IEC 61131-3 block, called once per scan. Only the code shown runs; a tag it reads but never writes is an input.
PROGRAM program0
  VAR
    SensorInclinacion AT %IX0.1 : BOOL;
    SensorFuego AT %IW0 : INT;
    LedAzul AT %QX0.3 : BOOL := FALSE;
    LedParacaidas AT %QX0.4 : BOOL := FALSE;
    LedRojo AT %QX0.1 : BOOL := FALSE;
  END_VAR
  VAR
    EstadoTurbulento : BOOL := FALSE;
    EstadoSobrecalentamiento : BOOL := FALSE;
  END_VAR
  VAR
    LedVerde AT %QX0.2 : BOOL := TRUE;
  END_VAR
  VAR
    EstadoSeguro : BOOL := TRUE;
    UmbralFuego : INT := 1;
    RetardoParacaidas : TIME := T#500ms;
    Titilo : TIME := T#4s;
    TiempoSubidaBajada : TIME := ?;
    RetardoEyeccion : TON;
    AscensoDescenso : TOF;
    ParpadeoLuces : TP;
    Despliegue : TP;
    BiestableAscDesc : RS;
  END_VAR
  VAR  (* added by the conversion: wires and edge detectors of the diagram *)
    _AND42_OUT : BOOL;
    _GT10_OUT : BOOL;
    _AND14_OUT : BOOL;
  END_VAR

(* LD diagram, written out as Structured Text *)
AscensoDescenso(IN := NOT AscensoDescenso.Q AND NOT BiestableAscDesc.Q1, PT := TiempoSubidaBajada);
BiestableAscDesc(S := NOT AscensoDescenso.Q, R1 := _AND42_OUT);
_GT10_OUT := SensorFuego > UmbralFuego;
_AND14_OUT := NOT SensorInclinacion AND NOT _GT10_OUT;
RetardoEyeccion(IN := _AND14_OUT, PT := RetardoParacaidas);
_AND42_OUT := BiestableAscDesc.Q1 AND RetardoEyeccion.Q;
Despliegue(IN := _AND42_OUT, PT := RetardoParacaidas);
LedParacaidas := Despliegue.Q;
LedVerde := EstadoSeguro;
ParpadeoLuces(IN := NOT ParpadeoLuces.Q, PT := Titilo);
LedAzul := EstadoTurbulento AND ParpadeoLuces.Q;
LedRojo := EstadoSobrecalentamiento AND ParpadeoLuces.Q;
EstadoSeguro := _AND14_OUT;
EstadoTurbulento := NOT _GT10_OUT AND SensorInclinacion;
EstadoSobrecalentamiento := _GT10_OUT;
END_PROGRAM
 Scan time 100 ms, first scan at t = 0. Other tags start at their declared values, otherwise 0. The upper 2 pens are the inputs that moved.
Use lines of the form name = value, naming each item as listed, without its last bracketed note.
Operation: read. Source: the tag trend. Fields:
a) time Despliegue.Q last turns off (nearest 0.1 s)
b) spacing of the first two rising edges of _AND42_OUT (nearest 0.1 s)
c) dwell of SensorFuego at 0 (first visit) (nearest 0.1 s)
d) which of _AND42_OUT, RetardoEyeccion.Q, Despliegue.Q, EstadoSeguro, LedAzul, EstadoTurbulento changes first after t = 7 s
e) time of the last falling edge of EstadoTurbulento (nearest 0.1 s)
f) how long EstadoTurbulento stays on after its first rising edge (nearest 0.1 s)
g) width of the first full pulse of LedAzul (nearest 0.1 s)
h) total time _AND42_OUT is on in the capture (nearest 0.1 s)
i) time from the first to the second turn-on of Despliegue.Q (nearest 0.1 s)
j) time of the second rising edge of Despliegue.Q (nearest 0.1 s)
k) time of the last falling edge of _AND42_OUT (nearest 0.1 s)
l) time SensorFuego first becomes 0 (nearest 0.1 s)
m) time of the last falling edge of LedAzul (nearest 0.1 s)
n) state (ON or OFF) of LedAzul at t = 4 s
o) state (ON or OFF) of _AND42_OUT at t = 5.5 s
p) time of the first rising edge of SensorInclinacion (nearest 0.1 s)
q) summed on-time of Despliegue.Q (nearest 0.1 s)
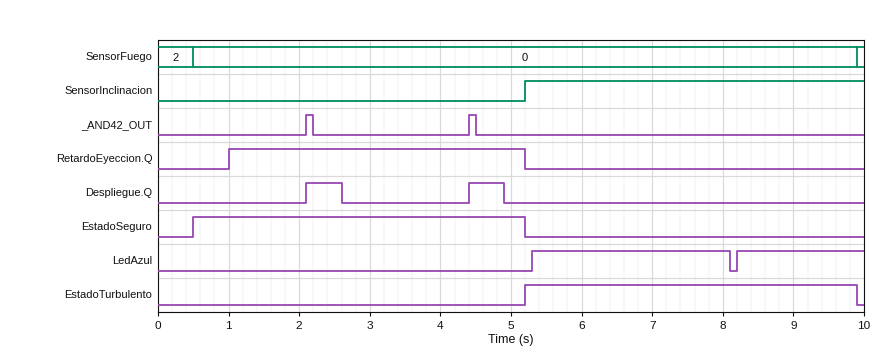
time Despliegue.Q last turns off = 4.9 s
spacing of the first two rising edges of _AND42_OUT = 2.3 s
dwell of SensorFuego at 0 (first visit) = 9.4 s
which of _AND42_OUT, RetardoEyeccion.Q, Despliegue.Q, EstadoSeguro, LedAzul, EstadoTurbulento changes first after t = 7 s = LedAzul
time of the last falling edge of EstadoTurbulento = 9.9 s
how long EstadoTurbulento stays on after its first rising edge = 4.7 s
width of the first full pulse of LedAzul = 2.8 s
total time _AND42_OUT is on in the capture = 0.2 s
time from the first to the second turn-on of Despliegue.Q = 2.3 s
time of the second rising edge of Despliegue.Q = 4.4 s
time of the last falling edge of _AND42_OUT = 4.5 s
time SensorFuego first becomes 0 = 0.5 s
time of the last falling edge of LedAzul = 8.1 s
state (ON or OFF) of LedAzul at t = 4 s = OFF
state (ON or OFF) of _AND42_OUT at t = 5.5 s = OFF
time of the first rising edge of SensorInclinacion = 5.2 s
summed on-time of Despliegue.Q = 1.0 s
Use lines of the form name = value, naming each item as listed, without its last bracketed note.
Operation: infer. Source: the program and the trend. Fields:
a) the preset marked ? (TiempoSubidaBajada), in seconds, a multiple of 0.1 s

the preset marked ? (TiempoSubidaBajada), in seconds, a multiple of 0.1 s = 2.0 s
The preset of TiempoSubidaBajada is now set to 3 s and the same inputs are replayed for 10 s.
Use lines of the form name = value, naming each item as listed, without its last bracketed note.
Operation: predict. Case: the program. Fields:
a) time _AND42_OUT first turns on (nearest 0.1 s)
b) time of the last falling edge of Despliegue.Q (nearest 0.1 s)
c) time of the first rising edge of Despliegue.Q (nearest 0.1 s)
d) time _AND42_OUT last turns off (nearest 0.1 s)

time _AND42_OUT first turns on = 3.1 s
time of the last falling edge of Despliegue.Q = 3.6 s
time of the first rising edge of Despliegue.Q = 3.1 s
time _AND42_OUT last turns off = 3.2 s
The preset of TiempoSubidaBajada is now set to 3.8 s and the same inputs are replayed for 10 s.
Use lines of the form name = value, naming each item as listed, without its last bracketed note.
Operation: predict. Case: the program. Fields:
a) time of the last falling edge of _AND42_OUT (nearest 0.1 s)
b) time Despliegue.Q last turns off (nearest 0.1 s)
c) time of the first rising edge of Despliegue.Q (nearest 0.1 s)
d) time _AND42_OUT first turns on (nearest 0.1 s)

time of the last falling edge of _AND42_OUT = 4.0 s
time Despliegue.Q last turns off = 4.4 s
time of the first rising edge of Despliegue.Q = 3.9 s
time _AND42_OUT first turns on = 3.9 s
